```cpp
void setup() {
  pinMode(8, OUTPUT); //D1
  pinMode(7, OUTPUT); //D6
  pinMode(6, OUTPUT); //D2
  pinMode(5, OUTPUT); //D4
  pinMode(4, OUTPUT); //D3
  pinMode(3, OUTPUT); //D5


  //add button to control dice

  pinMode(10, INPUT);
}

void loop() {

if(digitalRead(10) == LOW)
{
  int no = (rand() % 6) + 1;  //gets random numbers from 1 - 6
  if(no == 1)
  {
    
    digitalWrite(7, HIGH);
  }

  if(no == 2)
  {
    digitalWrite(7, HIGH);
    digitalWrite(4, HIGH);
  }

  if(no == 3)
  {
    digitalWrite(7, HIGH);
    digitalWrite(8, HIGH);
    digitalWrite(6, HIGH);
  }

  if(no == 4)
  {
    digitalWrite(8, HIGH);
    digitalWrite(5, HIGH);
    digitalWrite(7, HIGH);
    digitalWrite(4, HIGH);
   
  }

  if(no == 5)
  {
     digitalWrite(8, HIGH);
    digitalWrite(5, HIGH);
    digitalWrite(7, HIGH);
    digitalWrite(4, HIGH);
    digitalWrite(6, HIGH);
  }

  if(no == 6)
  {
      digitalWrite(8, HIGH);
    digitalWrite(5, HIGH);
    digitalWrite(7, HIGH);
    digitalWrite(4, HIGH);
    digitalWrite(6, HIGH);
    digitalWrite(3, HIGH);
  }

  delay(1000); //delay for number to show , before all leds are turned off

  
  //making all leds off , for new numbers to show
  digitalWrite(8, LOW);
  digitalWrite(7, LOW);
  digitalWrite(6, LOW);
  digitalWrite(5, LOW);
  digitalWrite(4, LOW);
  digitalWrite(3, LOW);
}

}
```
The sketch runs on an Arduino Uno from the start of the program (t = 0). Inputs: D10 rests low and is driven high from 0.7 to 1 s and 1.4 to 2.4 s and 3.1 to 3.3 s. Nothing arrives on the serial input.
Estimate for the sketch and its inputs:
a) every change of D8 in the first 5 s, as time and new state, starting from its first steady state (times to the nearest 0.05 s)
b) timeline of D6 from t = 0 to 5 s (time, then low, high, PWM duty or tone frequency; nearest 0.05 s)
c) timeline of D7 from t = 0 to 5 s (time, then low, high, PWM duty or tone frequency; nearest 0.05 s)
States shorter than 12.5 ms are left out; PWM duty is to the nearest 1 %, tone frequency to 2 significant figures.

0 s low; 1 s high; 2 s low; 2.4 s high; 3.4 s low; 4.4 s high
0 s low; 1 s high; 2 s low; 4.4 s high
0 s high; 2 s low; 2.4 s high
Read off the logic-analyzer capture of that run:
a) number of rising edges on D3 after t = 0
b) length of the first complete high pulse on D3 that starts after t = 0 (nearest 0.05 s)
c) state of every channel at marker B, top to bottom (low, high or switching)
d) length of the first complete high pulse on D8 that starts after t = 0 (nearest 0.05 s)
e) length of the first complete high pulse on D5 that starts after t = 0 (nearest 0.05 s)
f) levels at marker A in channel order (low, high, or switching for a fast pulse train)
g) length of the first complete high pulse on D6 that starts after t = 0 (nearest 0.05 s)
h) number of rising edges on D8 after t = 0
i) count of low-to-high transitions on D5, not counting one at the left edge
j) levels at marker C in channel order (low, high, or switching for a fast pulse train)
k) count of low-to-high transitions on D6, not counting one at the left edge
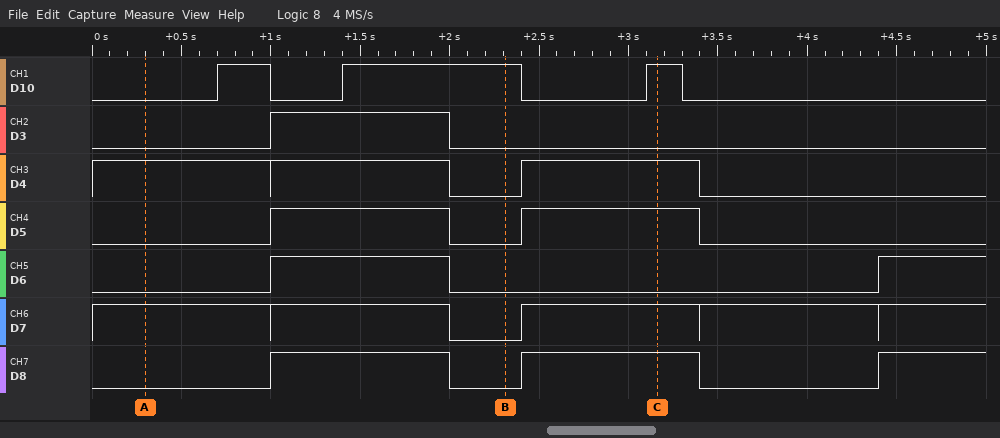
1
1.00 s
D10 high, D3 low, D4 low, D5 low, D6 low, D7 low, D8 low
1.00 s
1.00 s
D10 low, D3 low, D4 high, D5 low, D6 low, D7 high, D8 low
1.00 s
3
2
D10 high, D3 low, D4 high, D5 high, D6 low, D7 high, D8 high
2
